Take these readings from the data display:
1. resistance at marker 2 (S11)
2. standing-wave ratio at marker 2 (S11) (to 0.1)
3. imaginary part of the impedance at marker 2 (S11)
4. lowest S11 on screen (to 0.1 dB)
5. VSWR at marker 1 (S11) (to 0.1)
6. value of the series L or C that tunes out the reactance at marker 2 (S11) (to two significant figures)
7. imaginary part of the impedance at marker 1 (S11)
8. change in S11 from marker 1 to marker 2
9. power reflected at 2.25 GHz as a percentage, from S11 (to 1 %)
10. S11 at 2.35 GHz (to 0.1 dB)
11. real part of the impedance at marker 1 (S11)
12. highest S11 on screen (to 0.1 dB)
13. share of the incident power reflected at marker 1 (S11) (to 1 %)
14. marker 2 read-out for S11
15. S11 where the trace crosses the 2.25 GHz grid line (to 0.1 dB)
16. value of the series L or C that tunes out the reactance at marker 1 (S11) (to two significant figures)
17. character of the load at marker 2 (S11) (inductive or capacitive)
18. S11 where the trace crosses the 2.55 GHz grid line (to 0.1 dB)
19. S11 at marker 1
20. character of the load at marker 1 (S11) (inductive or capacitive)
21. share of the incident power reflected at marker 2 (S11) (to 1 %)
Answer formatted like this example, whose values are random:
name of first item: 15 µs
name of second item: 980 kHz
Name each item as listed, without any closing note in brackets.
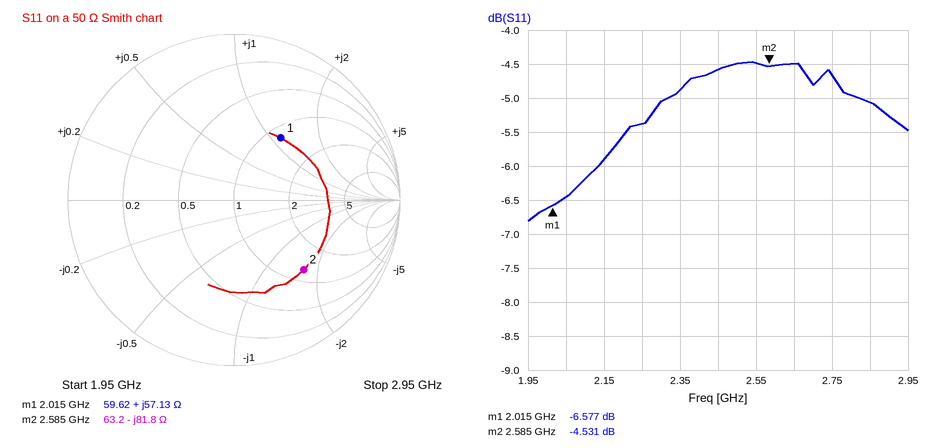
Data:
resistance at marker 2: 63.2 Ω
standing-wave ratio at marker 2 (S11): 3.9
imaginary part of the impedance at marker 2: -81.8 Ω
lowest S11 on screen: -6.8 dB
VSWR at marker 1 (S11): 2.8
value of the series L or C that tunes out the reactance at marker 2 (S11): 5.0 nH
imaginary part of the impedance at marker 1: +57.13 Ω
change in S11 from marker 1 to marker 2: 2.046 dB
power reflected at 2.25 GHz as a percentage, from S11: 29 %
S11 at 2.35 GHz: -4.9 dB
real part of the impedance at marker 1: 59.62 Ω
highest S11 on screen: -4.5 dB
share of the incident power reflected at marker 1 (S11): 22 %
marker 2 read-out for S11: -4.531 dB
S11 where the trace crosses the 2.25 GHz grid line: -5.4 dB
value of the series L or C that tunes out the reactance at marker 1 (S11): 1.4 pF
character of the load at marker 2 (S11): capacitive
S11 where the trace crosses the 2.55 GHz grid line: -4.5 dB
S11 at marker 1: -6.577 dB
character of the load at marker 1 (S11): inductive
share of the incident power reflected at marker 2 (S11): 35 %
